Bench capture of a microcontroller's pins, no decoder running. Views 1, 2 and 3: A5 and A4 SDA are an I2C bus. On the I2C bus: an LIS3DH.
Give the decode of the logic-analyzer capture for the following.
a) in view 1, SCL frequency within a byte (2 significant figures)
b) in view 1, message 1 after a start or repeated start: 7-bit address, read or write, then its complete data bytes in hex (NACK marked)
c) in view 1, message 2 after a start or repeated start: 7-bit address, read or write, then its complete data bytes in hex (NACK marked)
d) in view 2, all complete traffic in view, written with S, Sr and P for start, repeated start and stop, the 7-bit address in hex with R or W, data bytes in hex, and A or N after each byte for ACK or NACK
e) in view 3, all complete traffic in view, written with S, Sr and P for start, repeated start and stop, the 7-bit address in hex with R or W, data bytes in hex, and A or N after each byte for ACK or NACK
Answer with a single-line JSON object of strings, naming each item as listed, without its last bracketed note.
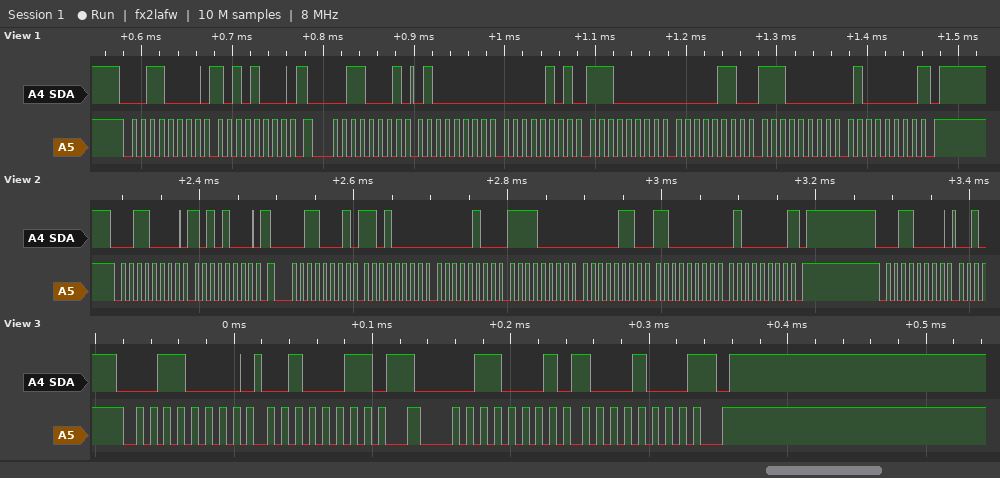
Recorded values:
{"in view 1, SCL frequency within a byte": "100 kHz", "in view 1, message 1 after a start or repeated start: 7-bit address, read or write, then its complete data bytes in hex": "0x18 write: A8", "in view 1, message 2 after a start or repeated start: 7-bit address, read or write, then its complete data bytes in hex": "0x18 read: 40 05 E0 06 E0 40 NACK", "in view 2, all complete traffic in view, written with S, Sr and P for start, repeated start and stop, the 7-bit address in hex with R or W, data bytes in hex, and A or N after each byte for ACK or NACK": "S 18W A A8 A Sr 18R A D0 A 04 A F0 A 06 A C0 A 40 N P S 18W A", "in view 3, all complete traffic in view, written with S, Sr and P for start, repeated start and stop, the 7-bit address in hex with R or W, data bytes in hex, and A or N after each byte for ACK or NACK": "S 18W A 23 A Sr 18R A 88 N P"}
